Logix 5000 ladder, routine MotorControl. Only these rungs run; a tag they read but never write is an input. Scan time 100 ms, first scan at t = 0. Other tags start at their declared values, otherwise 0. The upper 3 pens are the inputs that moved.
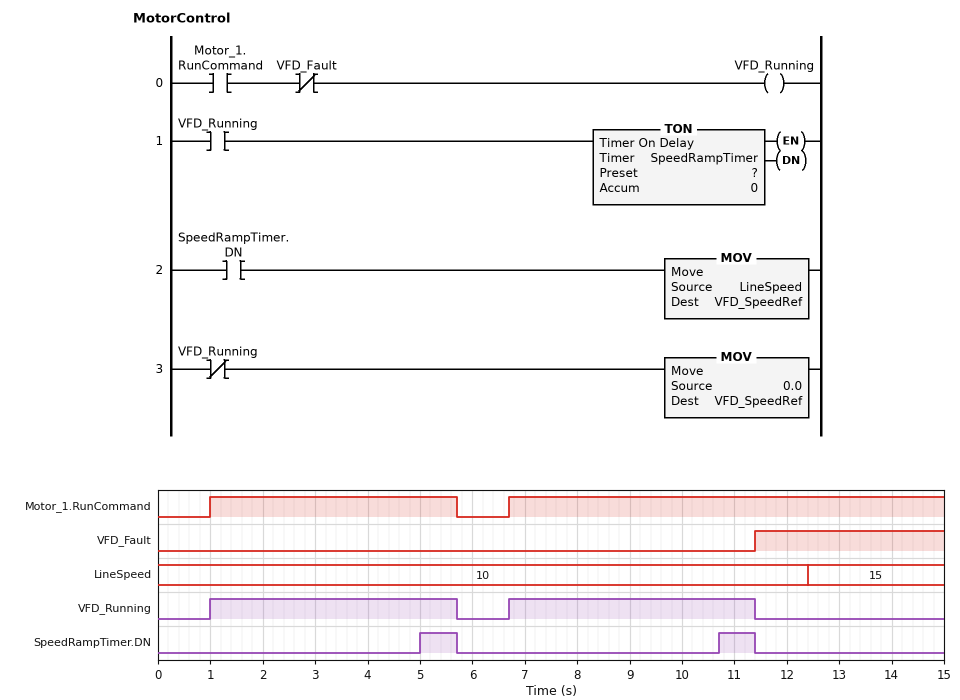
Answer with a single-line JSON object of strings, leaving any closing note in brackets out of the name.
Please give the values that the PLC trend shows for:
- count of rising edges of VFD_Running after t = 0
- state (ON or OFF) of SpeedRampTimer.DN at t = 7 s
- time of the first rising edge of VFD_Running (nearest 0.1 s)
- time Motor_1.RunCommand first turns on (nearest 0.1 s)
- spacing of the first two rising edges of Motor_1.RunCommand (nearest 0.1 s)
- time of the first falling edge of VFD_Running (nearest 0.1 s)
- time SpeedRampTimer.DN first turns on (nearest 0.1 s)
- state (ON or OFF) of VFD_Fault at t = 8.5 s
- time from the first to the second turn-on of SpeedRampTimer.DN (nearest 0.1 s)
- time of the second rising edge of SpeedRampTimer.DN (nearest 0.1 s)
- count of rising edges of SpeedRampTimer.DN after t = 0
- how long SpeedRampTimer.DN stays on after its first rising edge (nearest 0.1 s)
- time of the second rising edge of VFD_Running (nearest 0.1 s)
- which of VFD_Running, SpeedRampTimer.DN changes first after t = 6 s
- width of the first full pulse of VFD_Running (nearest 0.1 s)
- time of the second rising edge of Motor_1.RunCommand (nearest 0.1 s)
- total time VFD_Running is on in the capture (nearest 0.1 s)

{"count of rising edges of VFD_Running after t = 0": "2", "state (ON or OFF) of SpeedRampTimer.DN at t = 7 s": "OFF", "time of the first rising edge of VFD_Running": "1.0 s", "time Motor_1.RunCommand first turns on": "1.0 s", "spacing of the first two rising edges of Motor_1.RunCommand": "5.7 s", "time of the first falling edge of VFD_Running": "5.7 s", "time SpeedRampTimer.DN first turns on": "5.0 s", "state (ON or OFF) of VFD_Fault at t = 8.5 s": "OFF", "time from the first to the second turn-on of SpeedRampTimer.DN": "5.7 s", "time of the second rising edge of SpeedRampTimer.DN": "10.7 s", "count of rising edges of SpeedRampTimer.DN after t = 0": "2", "how long SpeedRampTimer.DN stays on after its first rising edge": "0.7 s", "time of the second rising edge of VFD_Running": "6.7 s", "which of VFD_Running, SpeedRampTimer.DN changes first after t = 6 s": "VFD_Running", "width of the first full pulse of VFD_Running": "4.7 s", "time of the second rising edge of Motor_1.RunCommand": "6.7 s", "total time VFD_Running is on in the capture": "9.4 s"}
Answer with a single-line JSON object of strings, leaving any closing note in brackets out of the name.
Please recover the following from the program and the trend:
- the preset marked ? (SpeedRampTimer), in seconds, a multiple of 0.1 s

{"the preset marked ? (SpeedRampTimer), in seconds, a multiple of 0.1 s": "4.0 s"}
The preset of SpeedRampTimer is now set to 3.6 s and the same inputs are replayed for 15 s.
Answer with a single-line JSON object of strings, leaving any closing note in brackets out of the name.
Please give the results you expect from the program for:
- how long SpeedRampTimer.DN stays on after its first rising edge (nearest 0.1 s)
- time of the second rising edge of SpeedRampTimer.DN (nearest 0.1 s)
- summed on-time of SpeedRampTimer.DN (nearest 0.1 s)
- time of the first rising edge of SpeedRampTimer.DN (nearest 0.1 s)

{"how long SpeedRampTimer.DN stays on after its first rising edge": "1.1 s", "time of the second rising edge of SpeedRampTimer.DN": "10.3 s", "summed on-time of SpeedRampTimer.DN": "2.2 s", "time of the first rising edge of SpeedRampTimer.DN": "4.6 s"}
